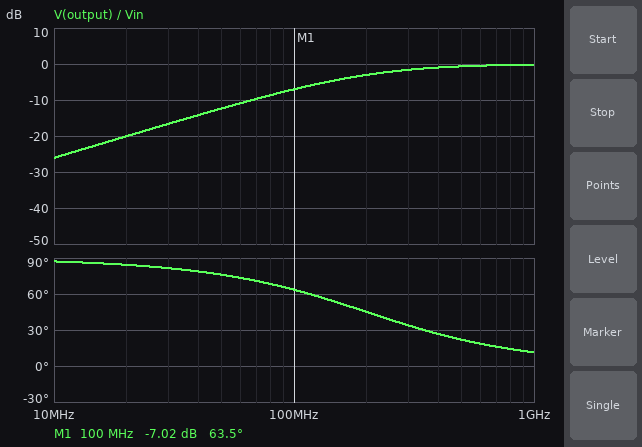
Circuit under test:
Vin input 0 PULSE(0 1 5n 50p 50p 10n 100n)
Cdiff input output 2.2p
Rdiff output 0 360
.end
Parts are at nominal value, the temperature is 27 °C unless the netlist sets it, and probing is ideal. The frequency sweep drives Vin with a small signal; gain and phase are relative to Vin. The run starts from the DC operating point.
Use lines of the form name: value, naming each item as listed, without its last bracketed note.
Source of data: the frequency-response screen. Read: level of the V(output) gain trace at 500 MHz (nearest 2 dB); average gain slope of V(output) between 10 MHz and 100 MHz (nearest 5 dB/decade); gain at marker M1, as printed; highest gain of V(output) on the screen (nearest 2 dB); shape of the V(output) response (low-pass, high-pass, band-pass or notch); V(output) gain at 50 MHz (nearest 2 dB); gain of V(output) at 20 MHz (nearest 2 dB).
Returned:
level of the V(output) gain trace at 500 MHz: 0 dB
average gain slope of V(output) between 10 MHz and 100 MHz: 20 dB/decade
gain at marker M1, as printed: -7.02 dB
highest gain of V(output) on the screen: 0 dB
shape of the V(output) response: high-pass
V(output) gain at 50 MHz: -12 dB
gain of V(output) at 20 MHz: -20 dB
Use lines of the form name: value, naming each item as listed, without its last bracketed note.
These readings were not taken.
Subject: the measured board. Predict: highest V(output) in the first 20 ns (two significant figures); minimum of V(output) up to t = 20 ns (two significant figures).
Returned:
highest V(output) in the first 20 ns: 970 mV
minimum of V(output) up to t = 20 ns: -970 mV
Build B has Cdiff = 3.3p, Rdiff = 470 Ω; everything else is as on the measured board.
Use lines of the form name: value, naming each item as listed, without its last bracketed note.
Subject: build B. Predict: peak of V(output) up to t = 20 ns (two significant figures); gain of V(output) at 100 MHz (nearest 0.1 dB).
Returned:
peak of V(output) up to t = 20 ns: 980 mV
gain of V(output) at 100 MHz: -3.1 dB
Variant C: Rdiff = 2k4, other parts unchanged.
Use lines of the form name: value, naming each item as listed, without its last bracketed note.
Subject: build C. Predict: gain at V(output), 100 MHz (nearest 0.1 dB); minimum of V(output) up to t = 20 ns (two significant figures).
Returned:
gain at V(output), 100 MHz: -0.4 dB
minimum of V(output) up to t = 20 ns: -850 mV
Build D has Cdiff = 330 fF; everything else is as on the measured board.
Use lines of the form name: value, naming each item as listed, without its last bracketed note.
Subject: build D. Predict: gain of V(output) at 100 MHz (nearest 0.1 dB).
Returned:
gain of V(output) at 100 MHz: -22.6 dB
